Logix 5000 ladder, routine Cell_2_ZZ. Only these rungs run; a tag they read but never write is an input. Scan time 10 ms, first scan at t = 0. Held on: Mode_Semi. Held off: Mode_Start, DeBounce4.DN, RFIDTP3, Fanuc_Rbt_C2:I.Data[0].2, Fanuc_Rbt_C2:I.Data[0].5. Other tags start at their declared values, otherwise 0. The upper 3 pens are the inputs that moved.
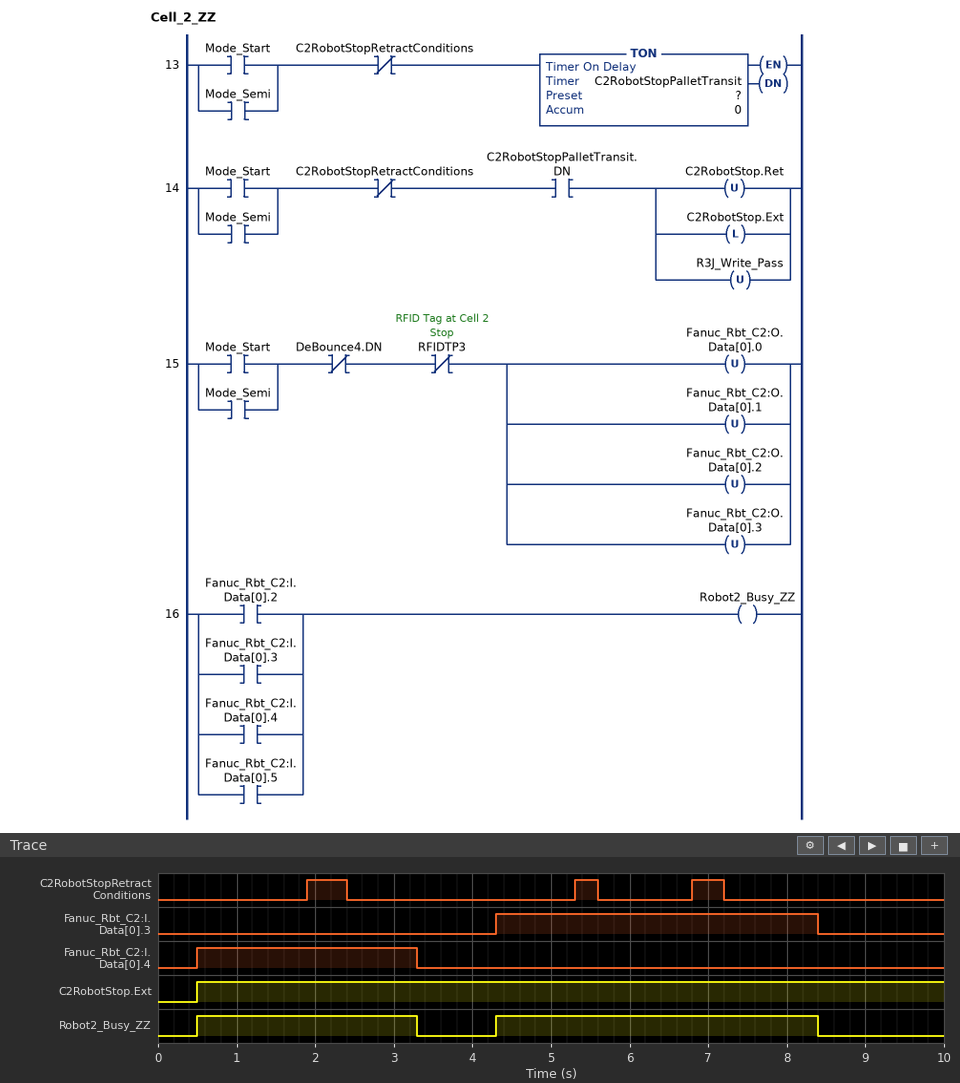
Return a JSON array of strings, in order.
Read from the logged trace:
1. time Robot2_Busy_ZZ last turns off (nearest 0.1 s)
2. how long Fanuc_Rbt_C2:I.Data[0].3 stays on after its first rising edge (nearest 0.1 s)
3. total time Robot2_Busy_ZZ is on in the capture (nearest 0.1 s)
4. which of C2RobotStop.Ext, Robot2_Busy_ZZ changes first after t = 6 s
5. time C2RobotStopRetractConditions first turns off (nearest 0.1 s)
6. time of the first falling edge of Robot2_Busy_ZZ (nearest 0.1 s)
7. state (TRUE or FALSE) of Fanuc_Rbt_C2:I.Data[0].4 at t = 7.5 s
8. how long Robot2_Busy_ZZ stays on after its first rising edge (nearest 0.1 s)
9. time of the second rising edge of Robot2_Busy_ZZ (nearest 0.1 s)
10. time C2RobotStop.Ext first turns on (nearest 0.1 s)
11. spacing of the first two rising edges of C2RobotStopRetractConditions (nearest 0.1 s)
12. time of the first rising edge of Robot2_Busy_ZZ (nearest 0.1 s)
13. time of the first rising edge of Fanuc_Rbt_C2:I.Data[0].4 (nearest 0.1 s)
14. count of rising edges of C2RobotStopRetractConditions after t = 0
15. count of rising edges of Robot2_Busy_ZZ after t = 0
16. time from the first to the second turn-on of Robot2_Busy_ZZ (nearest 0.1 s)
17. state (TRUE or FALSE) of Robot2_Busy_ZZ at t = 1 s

["8.4 s", "4.1 s", "6.9 s", "Robot2_Busy_ZZ", "2.4 s", "3.3 s", "FALSE", "2.8 s", "4.3 s", "0.5 s", "3.4 s", "0.5 s", "0.5 s", "3", "2", "3.8 s", "TRUE"]
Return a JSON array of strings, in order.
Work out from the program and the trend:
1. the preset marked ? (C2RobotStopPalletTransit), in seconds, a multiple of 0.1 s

["0.5 s"]
